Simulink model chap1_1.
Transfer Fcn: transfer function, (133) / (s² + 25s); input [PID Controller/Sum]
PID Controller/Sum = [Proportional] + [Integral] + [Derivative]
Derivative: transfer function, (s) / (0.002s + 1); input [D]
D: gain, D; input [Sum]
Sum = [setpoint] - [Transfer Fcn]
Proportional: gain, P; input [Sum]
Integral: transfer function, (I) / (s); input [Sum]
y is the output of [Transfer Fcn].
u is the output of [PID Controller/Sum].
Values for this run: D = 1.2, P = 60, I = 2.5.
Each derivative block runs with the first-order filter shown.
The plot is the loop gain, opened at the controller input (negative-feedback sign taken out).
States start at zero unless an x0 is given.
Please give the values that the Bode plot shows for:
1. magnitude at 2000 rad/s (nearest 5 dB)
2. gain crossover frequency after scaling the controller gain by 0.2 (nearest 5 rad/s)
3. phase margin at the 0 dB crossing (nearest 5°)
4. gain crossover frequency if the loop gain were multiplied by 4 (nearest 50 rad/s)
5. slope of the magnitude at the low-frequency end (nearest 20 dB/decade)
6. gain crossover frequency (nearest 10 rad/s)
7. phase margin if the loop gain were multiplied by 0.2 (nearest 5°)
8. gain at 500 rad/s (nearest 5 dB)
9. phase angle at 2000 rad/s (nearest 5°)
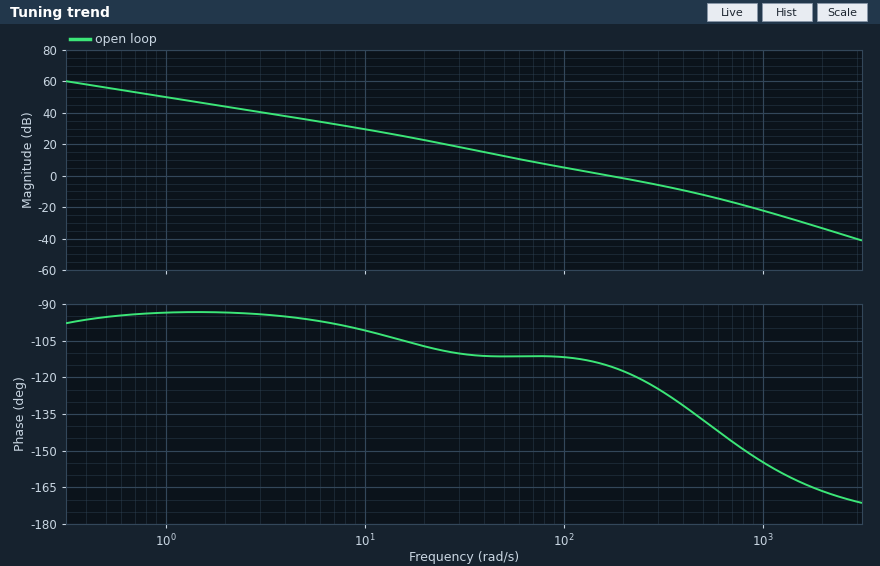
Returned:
-35 dB
45 rad/s
65°
500 rad/s
-20 dB/decade
170 rad/s
70°
-10 dB
-165°
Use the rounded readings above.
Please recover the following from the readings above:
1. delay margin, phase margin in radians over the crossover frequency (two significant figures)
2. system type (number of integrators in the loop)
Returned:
0.0067 s
1
